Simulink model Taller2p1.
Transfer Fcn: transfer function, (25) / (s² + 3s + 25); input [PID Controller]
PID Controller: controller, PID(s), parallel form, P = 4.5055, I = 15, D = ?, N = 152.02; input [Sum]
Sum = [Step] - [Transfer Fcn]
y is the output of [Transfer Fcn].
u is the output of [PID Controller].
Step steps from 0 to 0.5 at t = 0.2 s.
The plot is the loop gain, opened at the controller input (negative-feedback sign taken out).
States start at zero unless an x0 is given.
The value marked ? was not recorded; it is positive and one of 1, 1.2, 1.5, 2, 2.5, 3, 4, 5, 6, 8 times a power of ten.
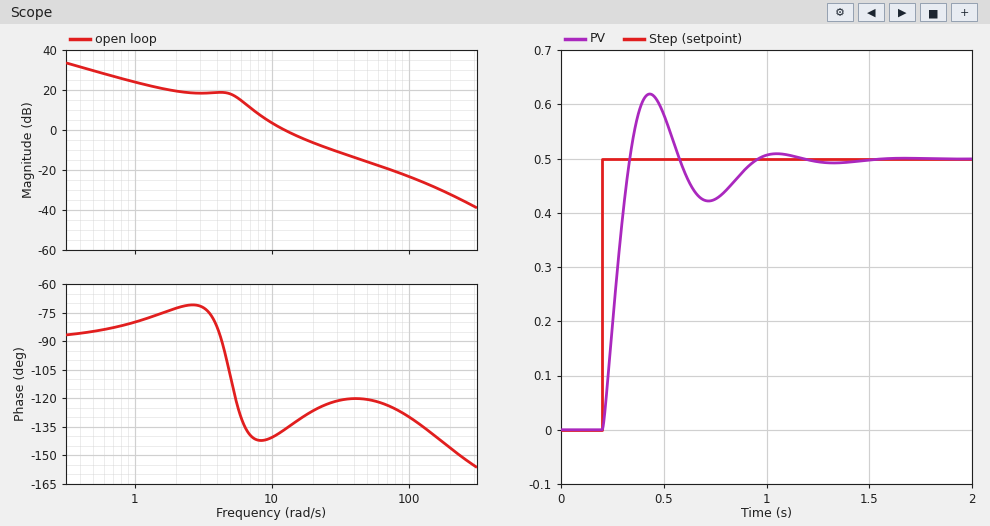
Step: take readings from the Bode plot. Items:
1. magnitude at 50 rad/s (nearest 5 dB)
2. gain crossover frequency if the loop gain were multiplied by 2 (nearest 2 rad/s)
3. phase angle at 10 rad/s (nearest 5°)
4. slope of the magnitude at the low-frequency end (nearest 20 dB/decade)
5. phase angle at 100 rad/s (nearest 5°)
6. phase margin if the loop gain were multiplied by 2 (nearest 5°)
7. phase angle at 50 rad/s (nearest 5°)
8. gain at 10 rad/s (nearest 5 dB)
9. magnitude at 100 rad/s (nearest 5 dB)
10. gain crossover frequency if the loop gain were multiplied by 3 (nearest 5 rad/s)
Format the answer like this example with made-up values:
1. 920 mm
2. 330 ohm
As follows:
1. -15 dB
2. 20 rad/s
3. -140°
4. -20 dB/decade
5. -130°
6. 55°
7. -120°
8. 5 dB
9. -25 dB
10. 25 rad/s
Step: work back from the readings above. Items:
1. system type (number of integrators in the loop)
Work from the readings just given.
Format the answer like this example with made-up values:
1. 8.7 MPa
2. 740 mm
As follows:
1. 1
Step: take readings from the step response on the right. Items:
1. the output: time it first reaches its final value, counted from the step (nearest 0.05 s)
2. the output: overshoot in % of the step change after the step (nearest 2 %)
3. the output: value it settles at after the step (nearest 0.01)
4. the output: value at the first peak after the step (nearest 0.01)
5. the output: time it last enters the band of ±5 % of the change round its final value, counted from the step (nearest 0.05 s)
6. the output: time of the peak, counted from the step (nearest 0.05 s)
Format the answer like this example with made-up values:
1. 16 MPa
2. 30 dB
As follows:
1. 0.15 s
2. 24 %
3. 0.50
4. 0.62
5. 0.70 s
6. 0.25 s
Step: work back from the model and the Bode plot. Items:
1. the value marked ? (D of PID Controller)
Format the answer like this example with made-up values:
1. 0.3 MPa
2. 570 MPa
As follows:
1. 0.3
